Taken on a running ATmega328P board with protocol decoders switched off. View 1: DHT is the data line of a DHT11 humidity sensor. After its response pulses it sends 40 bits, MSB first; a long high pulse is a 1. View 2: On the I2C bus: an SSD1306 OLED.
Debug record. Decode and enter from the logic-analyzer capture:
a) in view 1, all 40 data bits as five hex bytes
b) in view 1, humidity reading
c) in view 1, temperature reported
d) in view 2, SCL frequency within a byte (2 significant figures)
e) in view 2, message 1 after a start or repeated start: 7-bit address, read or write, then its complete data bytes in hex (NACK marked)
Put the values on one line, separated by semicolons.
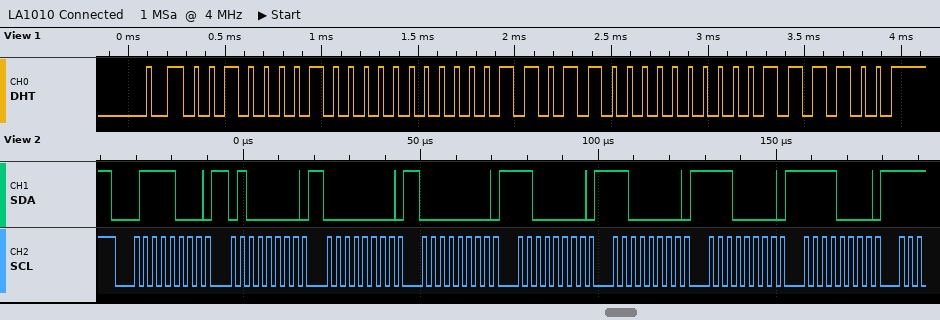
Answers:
21 00 1B 00 3C; 33 %; 27.0 °C; 400 kHz; 0x3C write: 40 00 00 C0 C0 E0 F0
